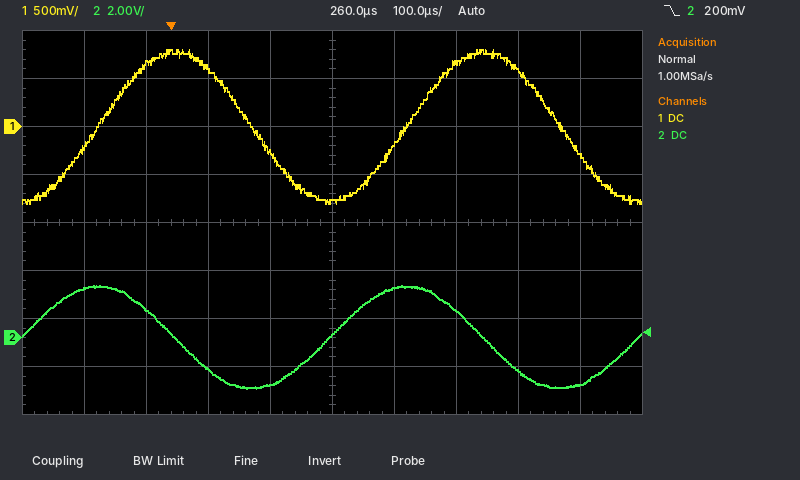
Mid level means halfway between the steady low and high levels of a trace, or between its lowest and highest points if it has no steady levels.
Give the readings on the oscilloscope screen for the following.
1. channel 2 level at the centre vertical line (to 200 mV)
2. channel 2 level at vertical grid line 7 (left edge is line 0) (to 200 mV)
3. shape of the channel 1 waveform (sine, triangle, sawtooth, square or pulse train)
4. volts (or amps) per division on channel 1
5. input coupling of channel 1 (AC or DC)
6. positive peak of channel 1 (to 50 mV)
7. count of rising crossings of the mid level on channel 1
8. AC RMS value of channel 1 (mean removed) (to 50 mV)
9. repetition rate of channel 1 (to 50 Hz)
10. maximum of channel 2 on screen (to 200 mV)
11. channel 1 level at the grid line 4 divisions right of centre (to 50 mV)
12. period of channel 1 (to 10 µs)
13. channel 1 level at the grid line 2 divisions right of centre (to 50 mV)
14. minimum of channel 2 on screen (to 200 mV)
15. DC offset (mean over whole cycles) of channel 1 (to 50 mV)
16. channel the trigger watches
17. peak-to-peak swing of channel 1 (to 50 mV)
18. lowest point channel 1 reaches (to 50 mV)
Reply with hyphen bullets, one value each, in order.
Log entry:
- 200 mV
- 1.2 V
- sine
- 500 mV
- DC
- 800 mV
- 2
- 550 mV
- 2.00 kHz
- 2.2 V
- -300 mV
- 500 µs
- 650 mV
- -2.2 V
- 0 mV
- channel 2
- 1.60 V
- -800 mV
